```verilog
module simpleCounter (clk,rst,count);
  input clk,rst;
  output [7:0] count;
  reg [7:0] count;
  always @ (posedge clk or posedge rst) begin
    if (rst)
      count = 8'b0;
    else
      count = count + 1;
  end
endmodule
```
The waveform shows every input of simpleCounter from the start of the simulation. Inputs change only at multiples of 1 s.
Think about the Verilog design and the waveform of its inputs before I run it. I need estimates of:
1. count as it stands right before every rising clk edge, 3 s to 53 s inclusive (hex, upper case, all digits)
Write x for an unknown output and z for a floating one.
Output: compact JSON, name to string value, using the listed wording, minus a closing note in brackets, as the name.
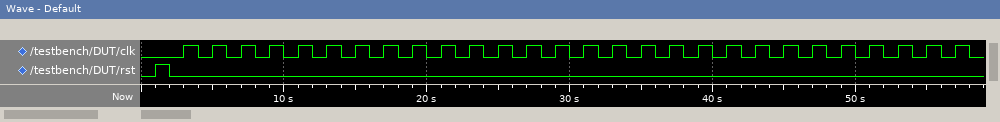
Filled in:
{"count as it stands right before every rising clk edge, 3 s to 53 s inclusive": "00, 01, 02, 03, 04, 05, 06, 07, 08, 09, 0A, 0B, 0C, 0D, 0E, 0F, 10, 11, 12, 13, 14, 15, 16, 17, 18, 19"}
